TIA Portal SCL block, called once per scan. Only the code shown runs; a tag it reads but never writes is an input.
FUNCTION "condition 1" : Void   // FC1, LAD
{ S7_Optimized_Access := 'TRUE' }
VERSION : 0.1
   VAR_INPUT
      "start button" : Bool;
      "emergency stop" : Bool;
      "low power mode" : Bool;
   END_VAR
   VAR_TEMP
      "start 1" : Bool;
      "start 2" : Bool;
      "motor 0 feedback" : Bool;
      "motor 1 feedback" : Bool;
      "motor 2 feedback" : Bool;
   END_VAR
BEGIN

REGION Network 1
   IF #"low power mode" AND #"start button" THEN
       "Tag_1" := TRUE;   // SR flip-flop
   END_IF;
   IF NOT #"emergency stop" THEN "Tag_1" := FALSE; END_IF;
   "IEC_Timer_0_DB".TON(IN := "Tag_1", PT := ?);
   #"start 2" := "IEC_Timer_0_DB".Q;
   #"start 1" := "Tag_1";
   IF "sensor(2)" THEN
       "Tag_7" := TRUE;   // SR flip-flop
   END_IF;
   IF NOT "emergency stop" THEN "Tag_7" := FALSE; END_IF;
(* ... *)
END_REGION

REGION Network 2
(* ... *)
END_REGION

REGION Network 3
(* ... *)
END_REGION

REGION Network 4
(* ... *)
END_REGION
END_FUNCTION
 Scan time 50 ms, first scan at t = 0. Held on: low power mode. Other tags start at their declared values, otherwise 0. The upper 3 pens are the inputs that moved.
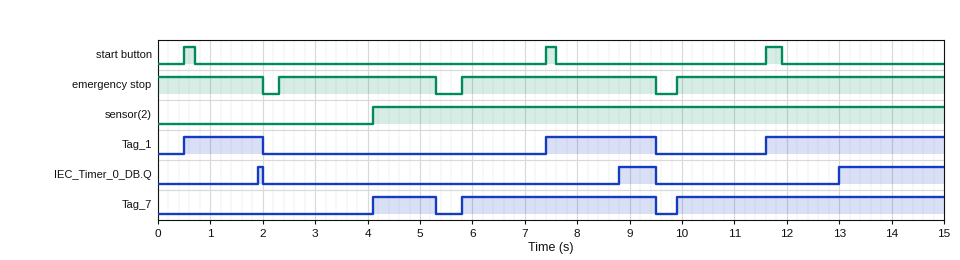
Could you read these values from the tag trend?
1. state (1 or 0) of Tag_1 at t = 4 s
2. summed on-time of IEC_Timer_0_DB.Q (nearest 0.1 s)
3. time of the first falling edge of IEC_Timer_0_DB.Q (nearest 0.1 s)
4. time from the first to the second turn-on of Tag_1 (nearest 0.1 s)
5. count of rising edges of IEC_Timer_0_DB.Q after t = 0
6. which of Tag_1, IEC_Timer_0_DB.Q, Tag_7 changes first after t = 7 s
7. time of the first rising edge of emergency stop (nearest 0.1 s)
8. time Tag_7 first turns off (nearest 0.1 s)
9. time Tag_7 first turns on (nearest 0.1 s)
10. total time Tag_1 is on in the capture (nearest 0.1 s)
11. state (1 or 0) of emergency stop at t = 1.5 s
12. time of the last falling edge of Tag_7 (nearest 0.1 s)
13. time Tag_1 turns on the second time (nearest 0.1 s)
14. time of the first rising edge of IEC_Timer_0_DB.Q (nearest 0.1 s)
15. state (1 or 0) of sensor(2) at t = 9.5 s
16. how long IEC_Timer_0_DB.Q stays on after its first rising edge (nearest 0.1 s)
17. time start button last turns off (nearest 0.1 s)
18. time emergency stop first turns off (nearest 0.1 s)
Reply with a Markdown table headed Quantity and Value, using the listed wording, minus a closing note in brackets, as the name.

| Quantity | Value |
|---|---|
| state (1 or 0) of Tag_1 at t = 4 s | 0 |
| summed on-time of IEC_Timer_0_DB.Q | 2.8 s |
| time of the first falling edge of IEC_Timer_0_DB.Q | 2.0 s |
| time from the first to the second turn-on of Tag_1 | 6.9 s |
| count of rising edges of IEC_Timer_0_DB.Q after t = 0 | 3 |
| which of Tag_1, IEC_Timer_0_DB.Q, Tag_7 changes first after t = 7 s | Tag_1 |
| time of the first rising edge of emergency stop | 2.3 s |
| time Tag_7 first turns off | 5.3 s |
| time Tag_7 first turns on | 4.1 s |
| total time Tag_1 is on in the capture | 7.0 s |
| state (1 or 0) of emergency stop at t = 1.5 s | 1 |
| time of the last falling edge of Tag_7 | 9.5 s |
| time Tag_1 turns on the second time | 7.4 s |
| time of the first rising edge of IEC_Timer_0_DB.Q | 1.9 s |
| state (1 or 0) of sensor(2) at t = 9.5 s | 1 |
| how long IEC_Timer_0_DB.Q stays on after its first rising edge | 0.1 s |
| time start button last turns off | 11.9 s |
| time emergency stop first turns off | 2.0 s |
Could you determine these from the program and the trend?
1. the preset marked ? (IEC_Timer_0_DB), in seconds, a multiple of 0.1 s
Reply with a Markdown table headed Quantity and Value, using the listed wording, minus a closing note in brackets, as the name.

| Quantity | Value |
|---|---|
| the preset marked ? (IEC_Timer_0_DB), in seconds, a multiple of 0.1 s | 1.4 s |
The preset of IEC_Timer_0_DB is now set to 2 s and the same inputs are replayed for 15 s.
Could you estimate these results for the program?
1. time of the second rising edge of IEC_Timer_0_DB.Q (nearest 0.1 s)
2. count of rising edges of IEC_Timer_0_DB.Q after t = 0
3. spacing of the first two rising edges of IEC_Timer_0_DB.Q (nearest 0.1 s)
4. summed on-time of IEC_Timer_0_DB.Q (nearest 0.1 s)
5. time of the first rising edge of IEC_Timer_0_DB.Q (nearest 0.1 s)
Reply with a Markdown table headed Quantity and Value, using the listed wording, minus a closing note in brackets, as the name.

| Quantity | Value |
|---|---|
| time of the second rising edge of IEC_Timer_0_DB.Q | 13.6 s |
| count of rising edges of IEC_Timer_0_DB.Q after t = 0 | 2 |
| spacing of the first two rising edges of IEC_Timer_0_DB.Q | 4.2 s |
| summed on-time of IEC_Timer_0_DB.Q | 1.5 s |
| time of the first rising edge of IEC_Timer_0_DB.Q | 9.4 s |
